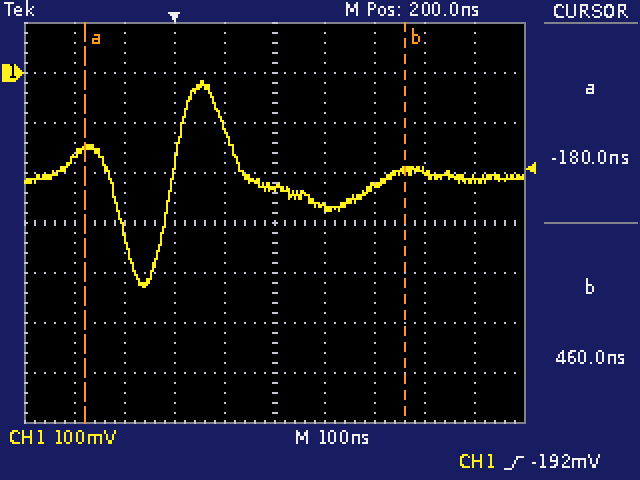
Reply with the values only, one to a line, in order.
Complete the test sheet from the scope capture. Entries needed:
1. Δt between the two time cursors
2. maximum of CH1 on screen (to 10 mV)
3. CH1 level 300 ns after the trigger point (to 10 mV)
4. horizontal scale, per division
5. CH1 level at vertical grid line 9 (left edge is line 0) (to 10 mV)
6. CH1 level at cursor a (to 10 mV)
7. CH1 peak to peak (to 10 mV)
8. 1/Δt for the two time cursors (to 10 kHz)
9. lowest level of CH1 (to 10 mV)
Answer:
640 ns
-20 mV
-270 mV
100 ns
-210 mV
-150 mV
410 mV
1.56 MHz
-430 mV
